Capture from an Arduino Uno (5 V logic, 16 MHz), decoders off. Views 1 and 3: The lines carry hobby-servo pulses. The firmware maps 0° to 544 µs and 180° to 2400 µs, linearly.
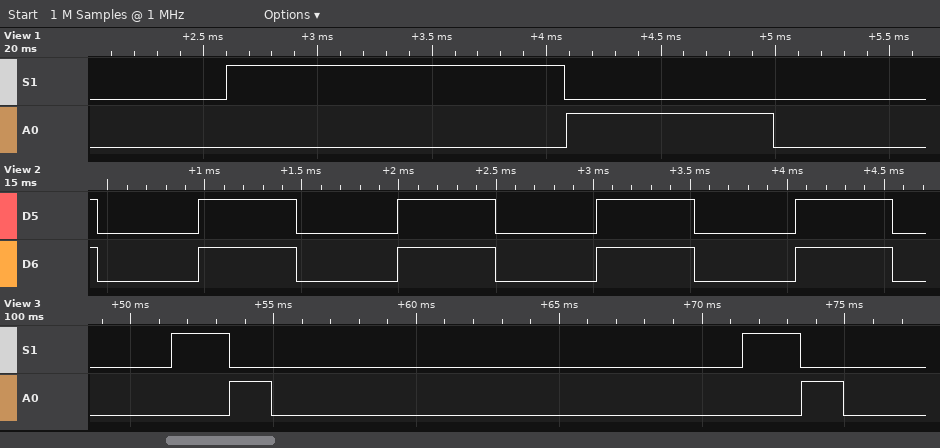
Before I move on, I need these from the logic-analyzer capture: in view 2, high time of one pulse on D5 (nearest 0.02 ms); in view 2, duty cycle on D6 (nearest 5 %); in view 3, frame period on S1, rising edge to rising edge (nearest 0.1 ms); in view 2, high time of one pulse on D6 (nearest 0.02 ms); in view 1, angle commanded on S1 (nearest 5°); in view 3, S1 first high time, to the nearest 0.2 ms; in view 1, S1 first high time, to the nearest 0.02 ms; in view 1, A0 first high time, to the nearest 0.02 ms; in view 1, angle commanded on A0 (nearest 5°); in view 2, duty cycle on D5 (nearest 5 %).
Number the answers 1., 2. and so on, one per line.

1. 0.50 ms
2. 50 %
3. 20.0 ms
4. 0.50 ms
5. 90°
6. 2.0 ms
7. 1.48 ms
8. 0.90 ms
9. 35°
10. 50 %
